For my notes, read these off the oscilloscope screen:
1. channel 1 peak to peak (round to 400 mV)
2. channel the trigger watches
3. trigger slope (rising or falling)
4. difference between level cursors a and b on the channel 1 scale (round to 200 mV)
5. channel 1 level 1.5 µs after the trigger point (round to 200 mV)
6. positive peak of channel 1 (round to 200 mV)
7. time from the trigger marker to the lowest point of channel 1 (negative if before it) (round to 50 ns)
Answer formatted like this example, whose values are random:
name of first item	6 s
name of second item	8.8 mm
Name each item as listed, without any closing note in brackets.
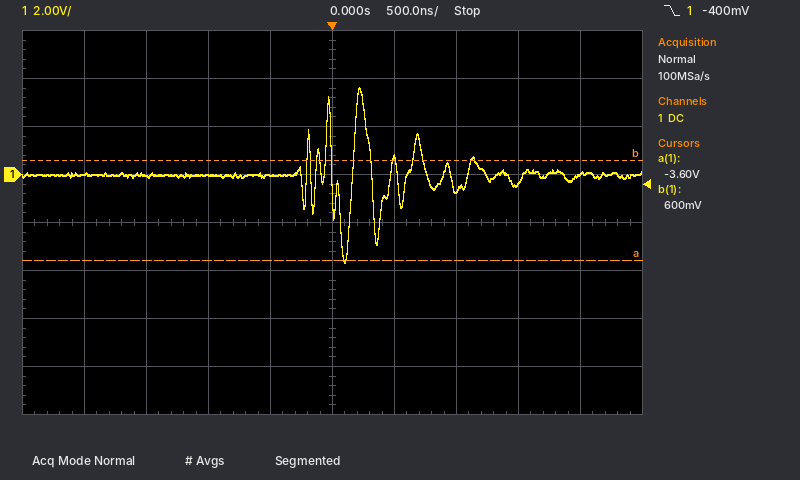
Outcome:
channel 1 peak to peak	7.2 V
channel the trigger watches	channel 1
trigger slope	falling
difference between level cursors a and b on the channel 1 scale	4.2 V
channel 1 level 1.5 µs after the trigger point	-400 mV
positive peak of channel 1	3.6 V
time from the trigger marker to the lowest point of channel 1 (negative if before it)	+100 ns
